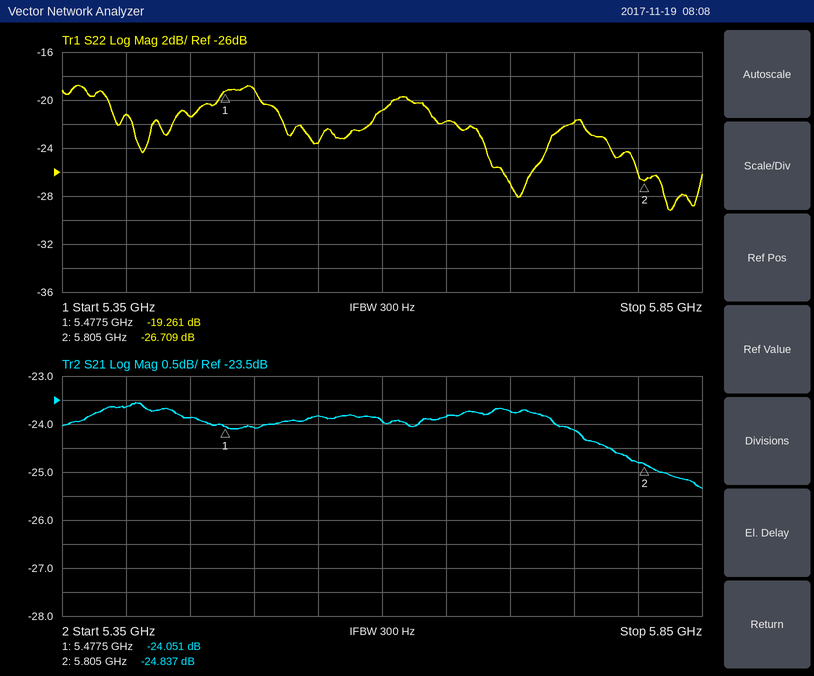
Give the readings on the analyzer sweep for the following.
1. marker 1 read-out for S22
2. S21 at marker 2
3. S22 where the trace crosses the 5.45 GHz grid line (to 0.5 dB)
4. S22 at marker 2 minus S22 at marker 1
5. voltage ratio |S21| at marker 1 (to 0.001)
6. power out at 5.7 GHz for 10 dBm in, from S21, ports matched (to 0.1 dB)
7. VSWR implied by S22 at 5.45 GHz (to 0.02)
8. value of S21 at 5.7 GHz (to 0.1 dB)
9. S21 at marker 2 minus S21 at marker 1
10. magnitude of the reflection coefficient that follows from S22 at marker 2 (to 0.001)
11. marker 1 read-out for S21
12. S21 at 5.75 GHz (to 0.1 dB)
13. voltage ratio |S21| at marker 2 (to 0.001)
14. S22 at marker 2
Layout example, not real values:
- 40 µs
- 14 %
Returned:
- -19.261 dB
- -24.837 dB
- -21.5 dB
- -7.448 dB
- 0.063
- -13.7 dBm
- 1.18
- -23.7 dB
- -0.786 dB
- 0.046
- -24.051 dB
- -24.1 dB
- 0.057
- -26.709 dB
